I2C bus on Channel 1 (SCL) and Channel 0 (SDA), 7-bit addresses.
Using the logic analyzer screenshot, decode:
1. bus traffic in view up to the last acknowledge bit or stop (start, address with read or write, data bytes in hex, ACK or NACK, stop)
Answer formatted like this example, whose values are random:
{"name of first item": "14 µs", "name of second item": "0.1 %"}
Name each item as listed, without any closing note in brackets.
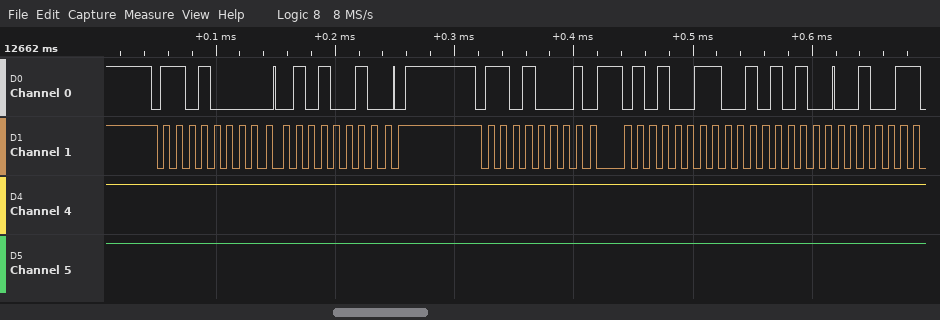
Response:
{"bus traffic in view up to the last acknowledge bit or stop": "start, address 68 write ACK, 52 ACK, stop, start, address 68 read ACK, 53 ACK, 54 ACK"}
